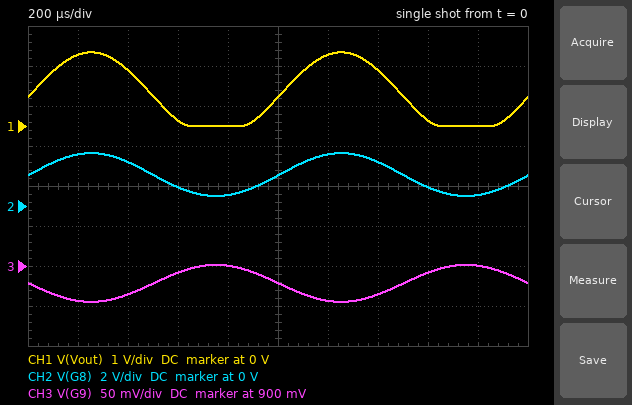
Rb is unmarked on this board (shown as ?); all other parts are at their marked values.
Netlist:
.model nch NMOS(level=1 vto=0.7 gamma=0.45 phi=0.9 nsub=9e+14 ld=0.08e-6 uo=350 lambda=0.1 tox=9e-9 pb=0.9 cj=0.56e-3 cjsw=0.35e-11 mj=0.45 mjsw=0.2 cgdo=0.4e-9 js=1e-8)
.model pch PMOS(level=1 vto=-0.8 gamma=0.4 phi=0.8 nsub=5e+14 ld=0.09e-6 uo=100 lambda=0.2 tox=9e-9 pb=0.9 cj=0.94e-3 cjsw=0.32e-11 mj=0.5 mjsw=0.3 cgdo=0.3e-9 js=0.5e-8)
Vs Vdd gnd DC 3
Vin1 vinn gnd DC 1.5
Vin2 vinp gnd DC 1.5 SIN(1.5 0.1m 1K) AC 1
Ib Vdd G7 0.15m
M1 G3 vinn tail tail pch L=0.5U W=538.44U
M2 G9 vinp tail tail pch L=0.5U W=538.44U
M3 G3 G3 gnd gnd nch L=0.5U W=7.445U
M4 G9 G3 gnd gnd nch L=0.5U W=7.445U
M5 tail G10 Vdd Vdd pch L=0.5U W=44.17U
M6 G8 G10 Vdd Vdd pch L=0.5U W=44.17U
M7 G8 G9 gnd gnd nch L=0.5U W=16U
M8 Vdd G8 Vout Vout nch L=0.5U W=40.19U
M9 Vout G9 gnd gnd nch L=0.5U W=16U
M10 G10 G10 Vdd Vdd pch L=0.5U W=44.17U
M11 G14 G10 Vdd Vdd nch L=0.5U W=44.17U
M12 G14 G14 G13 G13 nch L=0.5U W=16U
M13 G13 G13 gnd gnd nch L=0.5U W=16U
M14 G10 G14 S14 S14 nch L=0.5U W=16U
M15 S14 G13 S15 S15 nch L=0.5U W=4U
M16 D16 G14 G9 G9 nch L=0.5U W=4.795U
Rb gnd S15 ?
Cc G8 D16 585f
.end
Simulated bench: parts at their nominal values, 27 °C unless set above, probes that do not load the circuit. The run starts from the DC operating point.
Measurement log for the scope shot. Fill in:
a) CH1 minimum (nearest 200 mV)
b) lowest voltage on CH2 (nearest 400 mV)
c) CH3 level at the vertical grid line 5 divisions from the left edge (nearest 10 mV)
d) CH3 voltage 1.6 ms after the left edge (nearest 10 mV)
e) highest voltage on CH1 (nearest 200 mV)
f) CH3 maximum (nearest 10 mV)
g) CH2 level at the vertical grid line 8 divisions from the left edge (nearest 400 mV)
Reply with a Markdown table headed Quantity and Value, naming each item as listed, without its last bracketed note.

| Quantity | Value |
|---|---|
| CH1 minimum | 0 V |
| lowest voltage on CH2 | 400 mV |
| CH3 level at the vertical grid line 5 divisions from the left edge | 880 mV |
| CH3 voltage 1.6 ms after the left edge | 890 mV |
| highest voltage on CH1 | 1.8 V |
| CH3 maximum | 900 mV |
| CH2 level at the vertical grid line 8 divisions from the left edge | 800 mV |
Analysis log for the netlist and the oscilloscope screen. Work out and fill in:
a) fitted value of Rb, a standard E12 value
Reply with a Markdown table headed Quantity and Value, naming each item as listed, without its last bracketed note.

| Quantity | Value |
|---|---|
| fitted value of Rb, a standard E12 value | 1.2 kΩ |
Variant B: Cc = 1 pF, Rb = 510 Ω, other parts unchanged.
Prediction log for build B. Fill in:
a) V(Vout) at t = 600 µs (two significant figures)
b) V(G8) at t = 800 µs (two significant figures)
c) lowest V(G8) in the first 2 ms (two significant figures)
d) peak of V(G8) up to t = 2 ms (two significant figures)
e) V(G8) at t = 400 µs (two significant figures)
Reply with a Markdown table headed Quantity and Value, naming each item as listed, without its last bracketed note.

| Quantity | Value |
|---|---|
| V(Vout) at t = 600 µs | 280 mV |
| V(G8) at t = 800 µs | 810 mV |
| lowest V(G8) in the first 2 ms | 780 mV |
| peak of V(G8) up to t = 2 ms | 2.4 V |
| V(G8) at t = 400 µs | 2.0 V |
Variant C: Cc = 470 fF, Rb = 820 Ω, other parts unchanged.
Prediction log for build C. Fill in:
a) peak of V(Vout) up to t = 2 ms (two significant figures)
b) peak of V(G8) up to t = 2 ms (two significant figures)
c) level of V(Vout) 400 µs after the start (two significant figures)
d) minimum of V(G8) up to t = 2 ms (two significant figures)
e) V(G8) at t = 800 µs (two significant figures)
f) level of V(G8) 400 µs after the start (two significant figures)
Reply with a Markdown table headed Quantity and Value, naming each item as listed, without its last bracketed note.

| Quantity | Value |
|---|---|
| peak of V(Vout) up to t = 2 ms | 1.7 V |
| peak of V(G8) up to t = 2 ms | 2.5 V |
| level of V(Vout) 400 µs after the start | 1.3 V |
| minimum of V(G8) up to t = 2 ms | 650 mV |
| V(G8) at t = 800 µs | 690 mV |
| level of V(G8) 400 µs after the start | 2.1 V |
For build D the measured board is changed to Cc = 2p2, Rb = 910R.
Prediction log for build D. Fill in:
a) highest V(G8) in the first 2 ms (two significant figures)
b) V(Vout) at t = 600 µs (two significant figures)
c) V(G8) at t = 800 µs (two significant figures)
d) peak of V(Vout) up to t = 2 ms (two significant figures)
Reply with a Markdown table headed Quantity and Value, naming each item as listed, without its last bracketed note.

| Quantity | Value |
|---|---|
| highest V(G8) in the first 2 ms | 2.5 V |
| V(Vout) at t = 600 µs | 210 mV |
| V(G8) at t = 800 µs | 650 mV |
| peak of V(Vout) up to t = 2 ms | 1.7 V |
